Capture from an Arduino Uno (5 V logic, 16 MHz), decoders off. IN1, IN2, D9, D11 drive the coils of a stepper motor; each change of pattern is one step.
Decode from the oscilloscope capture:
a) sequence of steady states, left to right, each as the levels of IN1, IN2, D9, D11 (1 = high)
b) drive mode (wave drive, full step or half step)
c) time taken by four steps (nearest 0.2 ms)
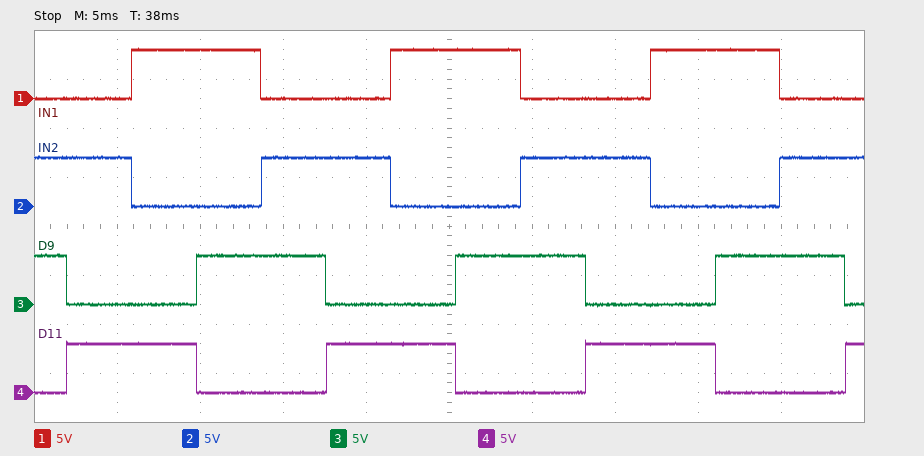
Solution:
0110 0101 1001 1010 0110 0101 1001 1010 0110 0101 1001 1010 0110 0101
full step
15.6 ms
